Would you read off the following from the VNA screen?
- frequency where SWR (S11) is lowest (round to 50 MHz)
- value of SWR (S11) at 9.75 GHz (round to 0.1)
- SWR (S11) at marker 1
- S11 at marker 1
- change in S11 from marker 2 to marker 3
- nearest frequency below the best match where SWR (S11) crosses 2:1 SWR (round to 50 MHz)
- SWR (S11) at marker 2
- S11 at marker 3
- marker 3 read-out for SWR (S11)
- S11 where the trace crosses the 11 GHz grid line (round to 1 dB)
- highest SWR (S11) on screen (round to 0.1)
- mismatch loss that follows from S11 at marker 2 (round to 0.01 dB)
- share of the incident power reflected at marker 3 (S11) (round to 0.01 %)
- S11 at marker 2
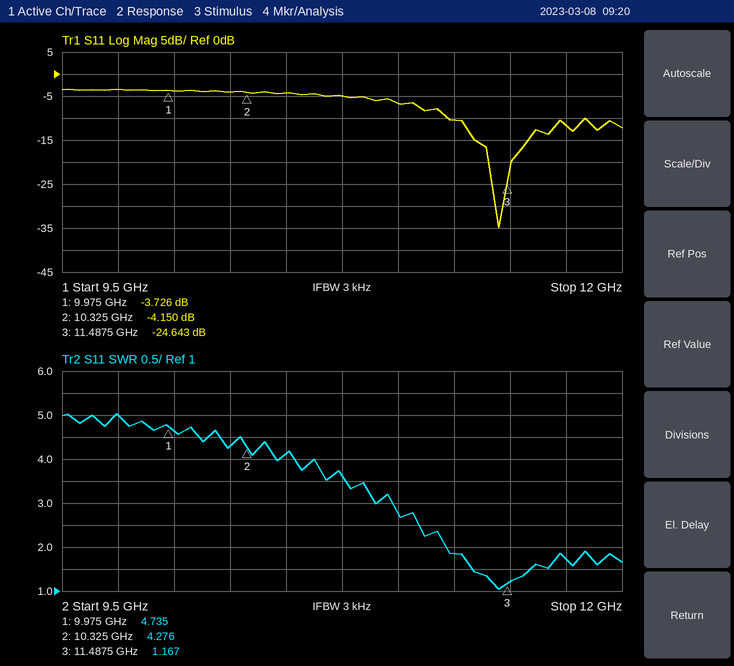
11.45 GHz
5.0
4.735
-3.726 dB
-20.493 dB
11.20 GHz
4.276
-24.643 dB
1.167
-7 dB
5.0
2.11 dB
0.34 %
-4.150 dB
